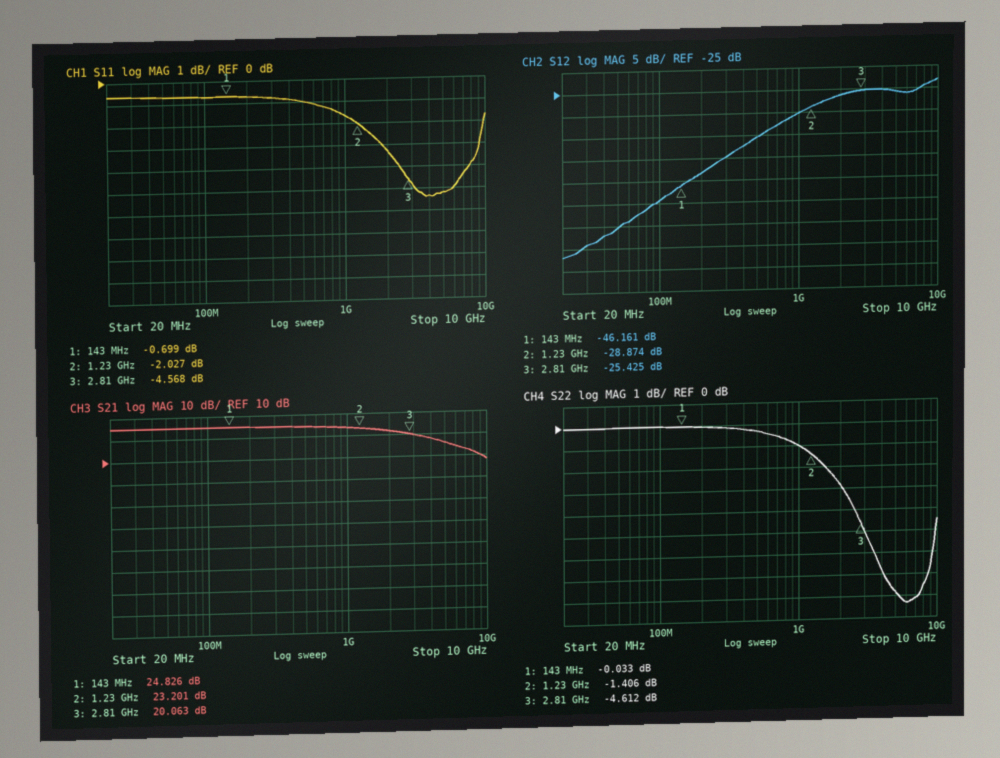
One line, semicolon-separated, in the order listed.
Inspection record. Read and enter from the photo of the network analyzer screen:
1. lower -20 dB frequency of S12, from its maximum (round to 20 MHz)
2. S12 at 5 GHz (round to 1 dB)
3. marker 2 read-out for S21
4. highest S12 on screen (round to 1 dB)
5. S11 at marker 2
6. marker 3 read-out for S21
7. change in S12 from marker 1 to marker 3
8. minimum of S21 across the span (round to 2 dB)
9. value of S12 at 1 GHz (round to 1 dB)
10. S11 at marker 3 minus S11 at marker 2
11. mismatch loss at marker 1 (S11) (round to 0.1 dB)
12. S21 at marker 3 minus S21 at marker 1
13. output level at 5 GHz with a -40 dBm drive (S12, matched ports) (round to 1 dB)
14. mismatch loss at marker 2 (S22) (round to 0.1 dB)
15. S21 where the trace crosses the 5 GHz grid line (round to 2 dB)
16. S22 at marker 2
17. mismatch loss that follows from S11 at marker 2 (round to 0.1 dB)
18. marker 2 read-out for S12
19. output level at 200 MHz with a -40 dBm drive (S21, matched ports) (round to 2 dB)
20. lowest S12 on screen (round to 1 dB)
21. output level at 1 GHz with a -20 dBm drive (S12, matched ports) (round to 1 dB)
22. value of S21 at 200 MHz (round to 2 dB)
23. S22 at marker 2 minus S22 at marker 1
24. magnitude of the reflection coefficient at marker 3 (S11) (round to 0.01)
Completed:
200 MHz; -26 dB; 23.201 dB; -23 dB; -2.027 dB; 20.063 dB; 20.736 dB; 8 dB; -30 dB; -2.541 dB; 8.3 dB; -4.763 dB; -66 dBm; 5.6 dB; 16 dB; -1.406 dB; 4.3 dB; -28.874 dB; -16 dBm; -62 dB; -50 dBm; 24 dB; -1.373 dB; 0.59
